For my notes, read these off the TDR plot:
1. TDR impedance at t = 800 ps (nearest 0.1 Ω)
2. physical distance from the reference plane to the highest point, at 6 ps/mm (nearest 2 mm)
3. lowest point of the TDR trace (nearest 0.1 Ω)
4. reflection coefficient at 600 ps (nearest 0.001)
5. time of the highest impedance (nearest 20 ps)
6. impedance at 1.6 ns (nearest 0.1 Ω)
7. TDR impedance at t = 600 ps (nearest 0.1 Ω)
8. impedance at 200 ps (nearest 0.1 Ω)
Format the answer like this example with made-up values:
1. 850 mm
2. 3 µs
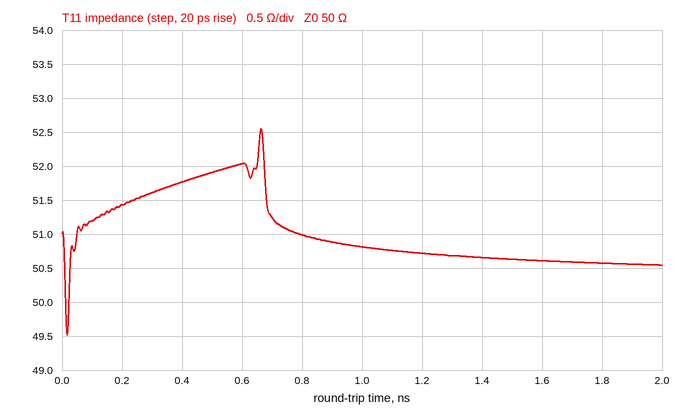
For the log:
1. 51.0 Ω
2. 56 mm
3. 49.5 Ω
4. +0.020
5. 660 ps
6. 50.6 Ω
7. 52.0 Ω
8. 51.4 Ω
